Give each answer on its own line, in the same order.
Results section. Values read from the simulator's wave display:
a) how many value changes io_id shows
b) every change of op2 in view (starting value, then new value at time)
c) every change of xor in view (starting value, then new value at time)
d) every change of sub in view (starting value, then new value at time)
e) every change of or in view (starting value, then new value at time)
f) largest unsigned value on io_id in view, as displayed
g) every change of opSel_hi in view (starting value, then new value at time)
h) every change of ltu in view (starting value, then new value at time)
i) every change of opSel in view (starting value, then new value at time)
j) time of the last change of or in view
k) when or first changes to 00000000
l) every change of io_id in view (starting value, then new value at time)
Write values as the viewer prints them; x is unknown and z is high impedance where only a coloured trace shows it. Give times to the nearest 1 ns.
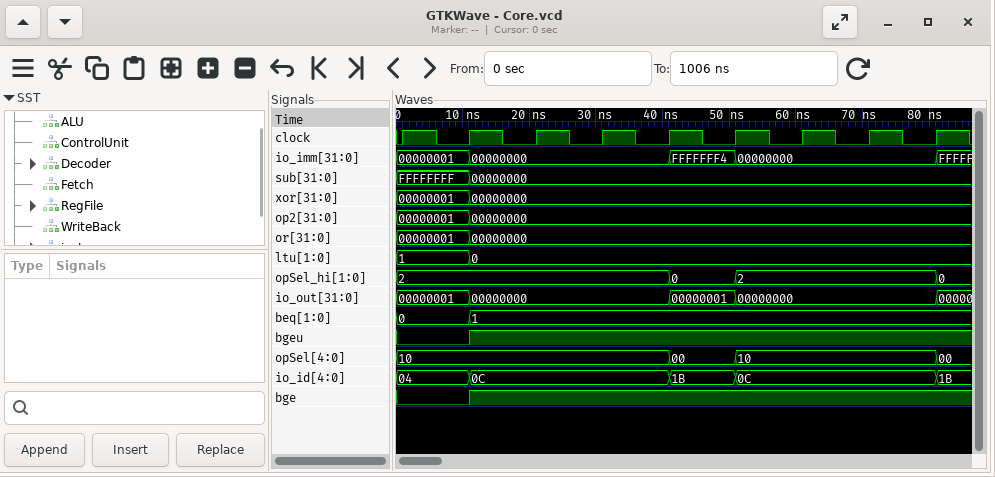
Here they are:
4
00000001, 00000000 at 11 ns
00000001, 00000000 at 11 ns
FFFFFFFF, 00000000 at 11 ns
00000001, 00000000 at 11 ns
1B
2, 0 at 41 ns, 2 at 51 ns, 0 at 81 ns
1, 0 at 11 ns
10, 00 at 41 ns, 10 at 51 ns, 00 at 81 ns
11 ns
11 ns
04, 0C at 11 ns, 1B at 41 ns, 0C at 51 ns, 1B at 81 ns
